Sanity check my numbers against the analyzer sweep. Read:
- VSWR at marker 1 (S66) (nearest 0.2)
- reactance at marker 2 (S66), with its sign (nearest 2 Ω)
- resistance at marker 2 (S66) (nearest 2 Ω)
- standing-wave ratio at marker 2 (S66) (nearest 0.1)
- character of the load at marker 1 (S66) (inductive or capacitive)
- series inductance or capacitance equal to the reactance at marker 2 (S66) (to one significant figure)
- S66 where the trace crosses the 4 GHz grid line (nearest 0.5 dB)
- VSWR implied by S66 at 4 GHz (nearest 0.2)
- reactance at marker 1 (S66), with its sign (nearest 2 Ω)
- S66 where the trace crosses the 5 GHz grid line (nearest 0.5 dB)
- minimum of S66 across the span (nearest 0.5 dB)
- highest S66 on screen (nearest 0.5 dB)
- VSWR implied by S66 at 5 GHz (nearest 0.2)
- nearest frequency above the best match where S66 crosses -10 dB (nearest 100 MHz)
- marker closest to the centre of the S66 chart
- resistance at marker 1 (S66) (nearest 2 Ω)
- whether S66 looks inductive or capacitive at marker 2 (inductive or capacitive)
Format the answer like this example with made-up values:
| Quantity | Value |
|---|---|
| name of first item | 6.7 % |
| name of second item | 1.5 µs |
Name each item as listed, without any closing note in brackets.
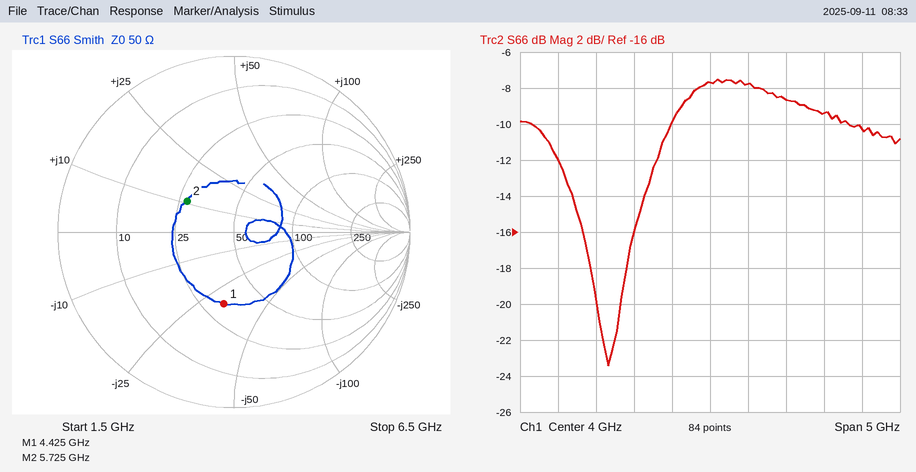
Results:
| Quantity | Value |
|---|---|
| VSWR at marker 1 (S66) | 2.4 |
| reactance at marker 2 (S66), with its sign | +10 Ω |
| resistance at marker 2 (S66) | 28 Ω |
| standing-wave ratio at marker 2 (S66) | 1.9 |
| character of the load at marker 1 (S66) | capacitive |
| series inductance or capacitance equal to the reactance at marker 2 (S66) | 300 pH |
| S66 where the trace crosses the 4 GHz grid line | -7.5 dB |
| VSWR implied by S66 at 4 GHz | 2.4 |
| reactance at marker 1 (S66), with its sign | -32 Ω |
| S66 where the trace crosses the 5 GHz grid line | -8.5 dB |
| minimum of S66 across the span | -23.5 dB |
| highest S66 on screen | -7.5 dB |
| VSWR implied by S66 at 5 GHz | 2.2 |
| nearest frequency above the best match where S66 crosses -10 dB | 3.5 GHz |
| marker closest to the centre of the S66 chart | marker 2 |
| resistance at marker 1 (S66) | 32 Ω |
| whether S66 looks inductive or capacitive at marker 2 | inductive |
